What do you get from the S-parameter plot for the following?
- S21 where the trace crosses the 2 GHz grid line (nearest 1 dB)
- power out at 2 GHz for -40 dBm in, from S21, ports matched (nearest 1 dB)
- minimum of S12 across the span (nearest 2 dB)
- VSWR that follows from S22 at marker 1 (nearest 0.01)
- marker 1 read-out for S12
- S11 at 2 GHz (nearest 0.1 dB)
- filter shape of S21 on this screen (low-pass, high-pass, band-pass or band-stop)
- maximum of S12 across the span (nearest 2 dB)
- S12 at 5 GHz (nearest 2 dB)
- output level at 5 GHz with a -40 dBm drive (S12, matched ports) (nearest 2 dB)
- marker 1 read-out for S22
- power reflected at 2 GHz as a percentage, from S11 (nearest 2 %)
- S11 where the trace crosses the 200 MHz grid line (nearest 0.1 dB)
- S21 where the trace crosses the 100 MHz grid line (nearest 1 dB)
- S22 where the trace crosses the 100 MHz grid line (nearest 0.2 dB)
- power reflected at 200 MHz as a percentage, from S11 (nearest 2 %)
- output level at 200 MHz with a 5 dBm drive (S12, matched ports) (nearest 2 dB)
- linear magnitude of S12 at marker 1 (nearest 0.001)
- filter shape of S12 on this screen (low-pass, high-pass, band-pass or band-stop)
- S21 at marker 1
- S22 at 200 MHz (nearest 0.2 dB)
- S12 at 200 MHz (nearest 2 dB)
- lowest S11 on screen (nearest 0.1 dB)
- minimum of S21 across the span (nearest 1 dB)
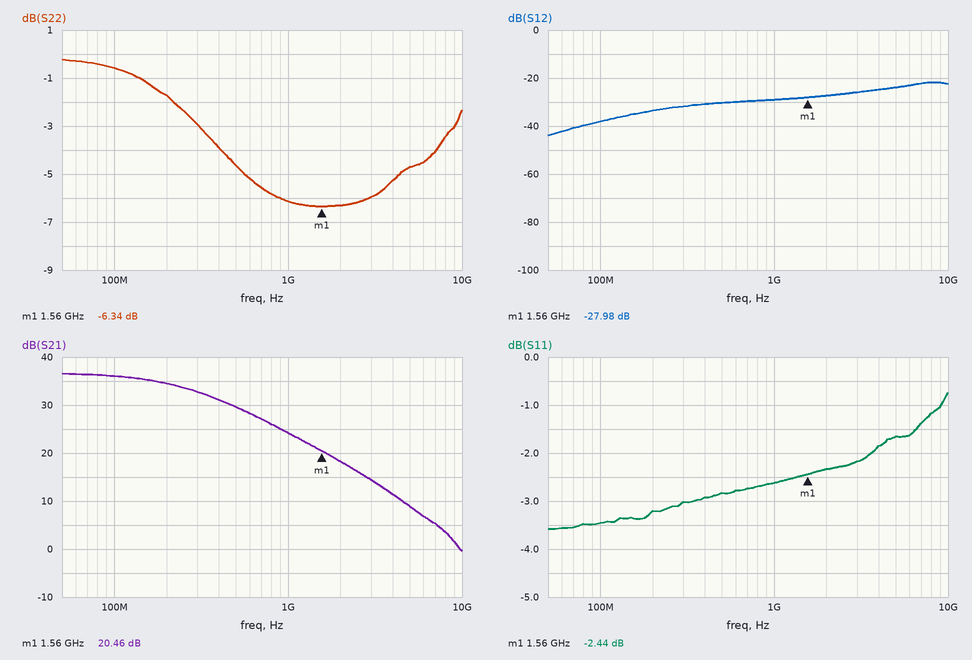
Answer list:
18 dB
-22 dBm
-44 dB
2.86
-27.98 dB
-2.3 dB
low-pass
-22 dB
-24 dB
-64 dBm
-6.34 dB
58 %
-3.2 dB
36 dB
-0.6 dB
48 %
-28 dBm
0.040
high-pass
20.46 dB
-1.8 dB
-34 dB
-3.6 dB
0 dB
